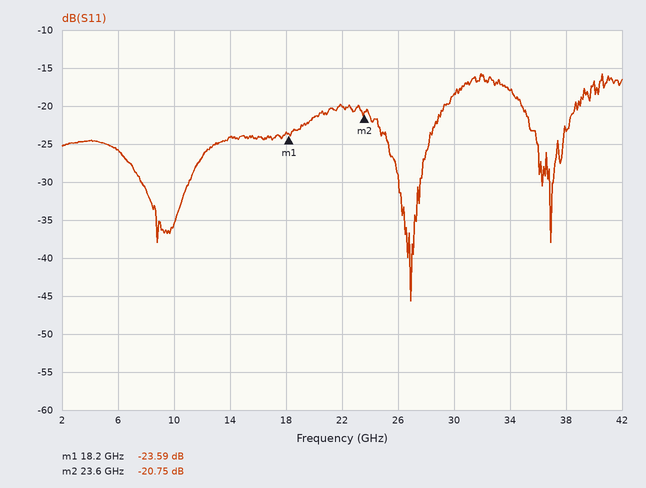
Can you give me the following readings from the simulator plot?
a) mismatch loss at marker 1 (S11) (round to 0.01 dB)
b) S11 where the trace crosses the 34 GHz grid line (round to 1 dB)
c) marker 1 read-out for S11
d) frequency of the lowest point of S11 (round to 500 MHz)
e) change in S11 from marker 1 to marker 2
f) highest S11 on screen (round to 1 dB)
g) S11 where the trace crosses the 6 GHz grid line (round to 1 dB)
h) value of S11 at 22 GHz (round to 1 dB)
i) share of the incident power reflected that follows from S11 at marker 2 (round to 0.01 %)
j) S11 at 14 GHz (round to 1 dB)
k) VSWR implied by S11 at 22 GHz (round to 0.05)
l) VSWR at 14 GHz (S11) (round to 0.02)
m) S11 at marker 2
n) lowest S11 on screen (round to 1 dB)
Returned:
0.02 dB
-18 dB
-23.59 dB
27.0 GHz
2.84 dB
-16 dB
-26 dB
-20 dB
0.84 %
-24 dB
1.20
1.14
-20.75 dB
-46 dB
